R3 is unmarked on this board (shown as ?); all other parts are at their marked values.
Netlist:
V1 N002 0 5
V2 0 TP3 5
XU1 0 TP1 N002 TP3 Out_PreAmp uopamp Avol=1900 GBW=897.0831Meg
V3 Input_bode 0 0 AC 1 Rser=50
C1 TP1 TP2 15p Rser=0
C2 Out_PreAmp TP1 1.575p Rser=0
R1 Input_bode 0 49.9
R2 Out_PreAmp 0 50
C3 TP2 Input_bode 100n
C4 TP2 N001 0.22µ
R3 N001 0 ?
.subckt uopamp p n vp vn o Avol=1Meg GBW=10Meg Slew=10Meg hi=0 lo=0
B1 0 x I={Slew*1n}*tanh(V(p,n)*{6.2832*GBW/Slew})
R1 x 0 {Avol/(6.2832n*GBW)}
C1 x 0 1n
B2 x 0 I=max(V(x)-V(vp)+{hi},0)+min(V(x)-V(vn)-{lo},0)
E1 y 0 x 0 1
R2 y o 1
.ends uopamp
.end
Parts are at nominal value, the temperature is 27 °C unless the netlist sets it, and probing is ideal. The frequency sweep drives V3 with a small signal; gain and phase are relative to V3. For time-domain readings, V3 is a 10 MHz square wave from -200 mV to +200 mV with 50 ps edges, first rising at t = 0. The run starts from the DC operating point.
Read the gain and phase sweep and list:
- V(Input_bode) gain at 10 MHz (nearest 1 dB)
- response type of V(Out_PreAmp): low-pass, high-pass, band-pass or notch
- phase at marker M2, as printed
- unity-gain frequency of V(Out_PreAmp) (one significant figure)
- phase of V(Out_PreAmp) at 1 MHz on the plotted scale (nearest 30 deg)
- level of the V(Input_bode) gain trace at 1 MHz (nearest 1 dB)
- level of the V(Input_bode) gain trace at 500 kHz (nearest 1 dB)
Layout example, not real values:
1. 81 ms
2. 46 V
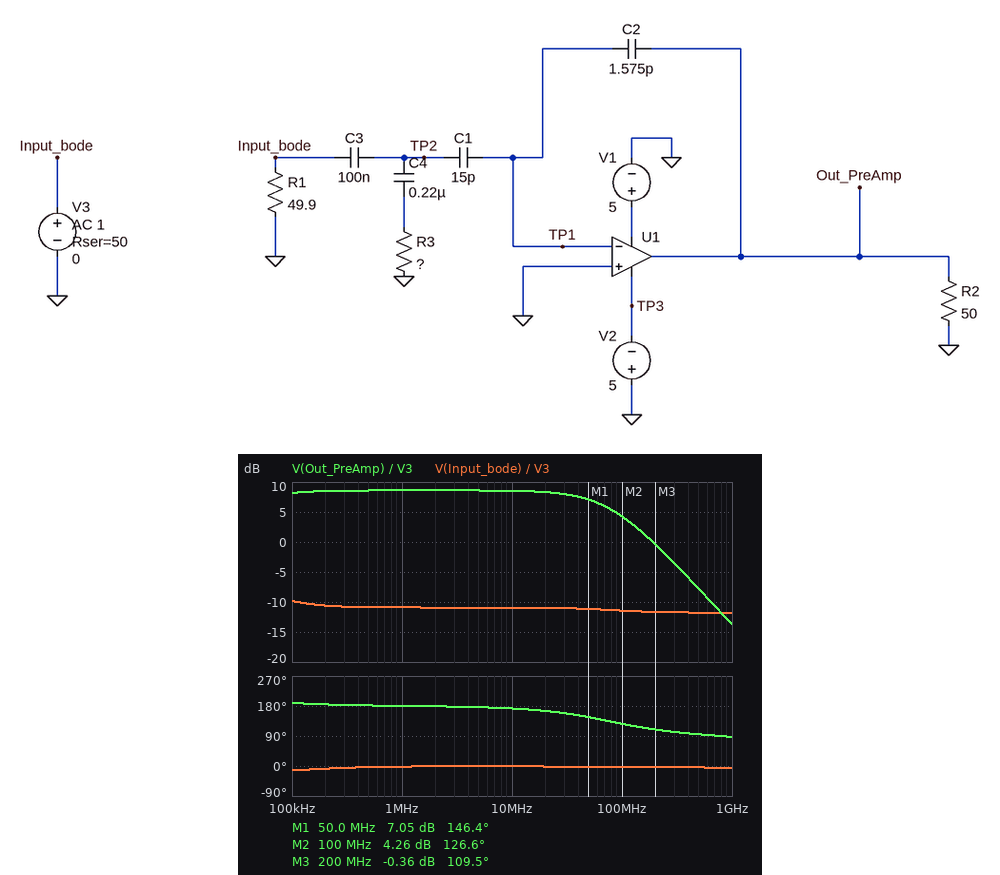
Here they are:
1. -11 dB
2. low-pass
3. 126.6 deg
4. 200 MHz
5. 180 deg
6. -11 dB
7. -11 dB
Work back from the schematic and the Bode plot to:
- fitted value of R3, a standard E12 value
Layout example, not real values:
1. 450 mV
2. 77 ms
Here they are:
1. 33 Ω
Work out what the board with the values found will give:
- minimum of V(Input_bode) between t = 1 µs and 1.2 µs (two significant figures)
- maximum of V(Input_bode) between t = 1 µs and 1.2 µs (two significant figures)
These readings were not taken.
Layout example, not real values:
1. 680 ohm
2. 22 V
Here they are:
1. -90 mV
2. 25 mV
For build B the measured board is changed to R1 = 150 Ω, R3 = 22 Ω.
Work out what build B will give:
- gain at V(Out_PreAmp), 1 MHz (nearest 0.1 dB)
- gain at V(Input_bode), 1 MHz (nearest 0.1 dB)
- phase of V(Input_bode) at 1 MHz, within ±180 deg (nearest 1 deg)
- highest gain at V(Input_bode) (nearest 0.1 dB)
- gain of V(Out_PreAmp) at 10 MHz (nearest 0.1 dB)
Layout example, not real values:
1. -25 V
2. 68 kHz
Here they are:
1. 8.4 dB
2. -11.1 dB
3. -4 deg
4. -2.5 dB
5. 8.3 dB
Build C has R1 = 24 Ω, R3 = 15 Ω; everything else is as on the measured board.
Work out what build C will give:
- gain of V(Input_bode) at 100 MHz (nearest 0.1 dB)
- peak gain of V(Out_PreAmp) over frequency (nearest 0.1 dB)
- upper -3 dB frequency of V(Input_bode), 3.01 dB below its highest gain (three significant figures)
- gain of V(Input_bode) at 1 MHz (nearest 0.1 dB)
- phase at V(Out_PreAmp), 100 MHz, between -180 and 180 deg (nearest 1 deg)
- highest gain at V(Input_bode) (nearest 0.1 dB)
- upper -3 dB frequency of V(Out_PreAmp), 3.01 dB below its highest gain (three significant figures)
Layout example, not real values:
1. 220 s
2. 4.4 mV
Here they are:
1. -16.4 dB
2. 3.4 dB
3. 101 kHz
4. -16.1 dB
5. 128 deg
6. -9.8 dB
7. 79.8 MHz
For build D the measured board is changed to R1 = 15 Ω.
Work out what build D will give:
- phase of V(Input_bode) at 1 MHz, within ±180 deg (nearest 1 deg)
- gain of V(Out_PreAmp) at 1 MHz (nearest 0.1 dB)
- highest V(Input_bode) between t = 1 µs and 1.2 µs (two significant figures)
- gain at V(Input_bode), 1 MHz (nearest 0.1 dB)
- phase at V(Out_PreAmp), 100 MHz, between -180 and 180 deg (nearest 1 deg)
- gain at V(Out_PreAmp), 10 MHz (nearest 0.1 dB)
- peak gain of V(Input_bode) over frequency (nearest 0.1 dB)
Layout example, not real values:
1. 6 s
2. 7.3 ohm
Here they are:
1. -1 deg
2. 4.2 dB
3. 26 mV
4. -15.3 dB
5. 128 deg
6. 4.1 dB
7. -12.7 dB
